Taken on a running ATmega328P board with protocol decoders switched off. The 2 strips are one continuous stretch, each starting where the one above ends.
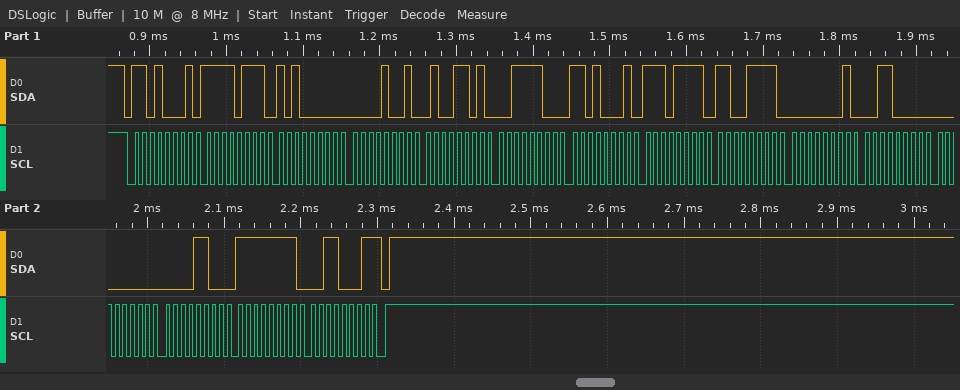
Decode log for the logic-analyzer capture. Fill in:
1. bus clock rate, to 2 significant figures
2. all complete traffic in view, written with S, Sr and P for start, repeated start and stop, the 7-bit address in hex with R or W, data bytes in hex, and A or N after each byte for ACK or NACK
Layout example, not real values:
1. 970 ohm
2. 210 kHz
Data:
1. 100 kHz
2. S 68R A F7 A A0 A 09 A 4D A 3C A D1 A EF A CF A 01 A 30 A 00 A 0C A FF A 31 N P
